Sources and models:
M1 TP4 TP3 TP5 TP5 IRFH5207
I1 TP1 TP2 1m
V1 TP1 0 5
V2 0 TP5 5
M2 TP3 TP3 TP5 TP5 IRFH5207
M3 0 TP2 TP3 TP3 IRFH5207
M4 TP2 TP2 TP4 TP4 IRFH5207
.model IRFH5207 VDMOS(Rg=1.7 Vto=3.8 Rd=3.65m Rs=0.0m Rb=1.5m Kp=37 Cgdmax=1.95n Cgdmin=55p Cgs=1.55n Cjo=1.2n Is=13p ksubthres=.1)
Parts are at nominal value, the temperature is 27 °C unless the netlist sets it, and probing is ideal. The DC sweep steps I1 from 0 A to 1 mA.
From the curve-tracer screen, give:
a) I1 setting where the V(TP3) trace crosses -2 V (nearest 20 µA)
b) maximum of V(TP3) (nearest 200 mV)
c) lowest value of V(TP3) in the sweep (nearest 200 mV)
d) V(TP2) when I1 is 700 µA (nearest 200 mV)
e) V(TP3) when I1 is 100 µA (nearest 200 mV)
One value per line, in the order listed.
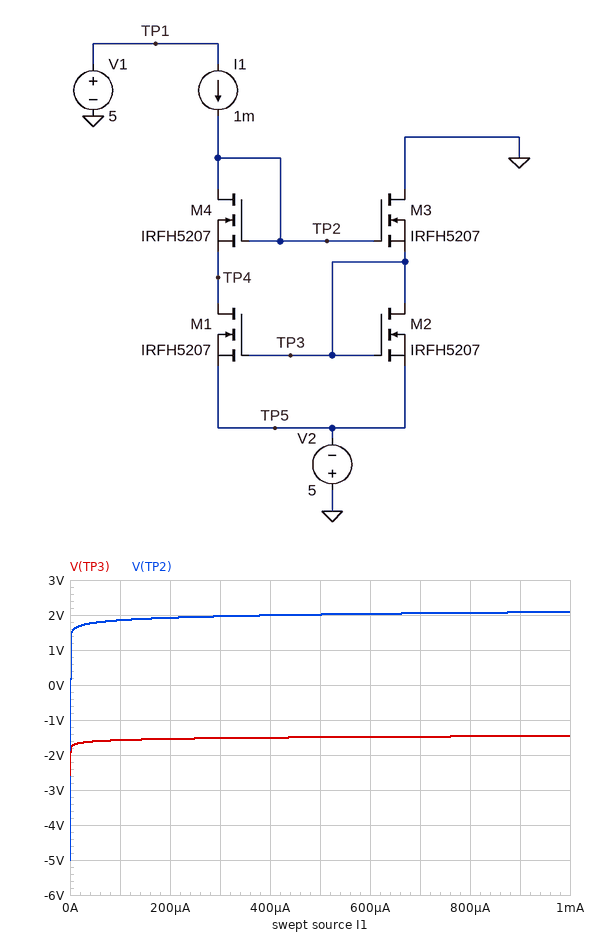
0 A
-1.4 V
-2.6 V
2.0 V
-1.6 V
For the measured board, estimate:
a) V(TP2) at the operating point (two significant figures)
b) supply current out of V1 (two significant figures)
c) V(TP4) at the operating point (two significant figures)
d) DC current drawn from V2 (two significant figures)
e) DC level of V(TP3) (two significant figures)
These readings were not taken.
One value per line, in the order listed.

2.1 V
1.0 mA
-1.5 V
2.0 mA
-1.5 V
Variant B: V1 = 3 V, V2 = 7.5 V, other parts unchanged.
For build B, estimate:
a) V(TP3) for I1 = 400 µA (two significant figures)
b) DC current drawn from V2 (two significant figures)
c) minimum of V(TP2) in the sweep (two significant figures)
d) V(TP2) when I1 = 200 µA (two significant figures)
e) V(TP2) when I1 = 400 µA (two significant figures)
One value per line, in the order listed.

-4.0 V
2.0 mA
-7.5 V
-580 mV
-510 mV
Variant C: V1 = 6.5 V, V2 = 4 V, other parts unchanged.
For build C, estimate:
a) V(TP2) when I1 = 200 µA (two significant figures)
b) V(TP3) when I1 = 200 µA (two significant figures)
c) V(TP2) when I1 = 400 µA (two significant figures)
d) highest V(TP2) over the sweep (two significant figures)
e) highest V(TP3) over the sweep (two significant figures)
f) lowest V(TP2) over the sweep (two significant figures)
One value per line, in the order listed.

2.9 V
-540 mV
3.0 V
3.1 V
-460 mV
-4.0 V
